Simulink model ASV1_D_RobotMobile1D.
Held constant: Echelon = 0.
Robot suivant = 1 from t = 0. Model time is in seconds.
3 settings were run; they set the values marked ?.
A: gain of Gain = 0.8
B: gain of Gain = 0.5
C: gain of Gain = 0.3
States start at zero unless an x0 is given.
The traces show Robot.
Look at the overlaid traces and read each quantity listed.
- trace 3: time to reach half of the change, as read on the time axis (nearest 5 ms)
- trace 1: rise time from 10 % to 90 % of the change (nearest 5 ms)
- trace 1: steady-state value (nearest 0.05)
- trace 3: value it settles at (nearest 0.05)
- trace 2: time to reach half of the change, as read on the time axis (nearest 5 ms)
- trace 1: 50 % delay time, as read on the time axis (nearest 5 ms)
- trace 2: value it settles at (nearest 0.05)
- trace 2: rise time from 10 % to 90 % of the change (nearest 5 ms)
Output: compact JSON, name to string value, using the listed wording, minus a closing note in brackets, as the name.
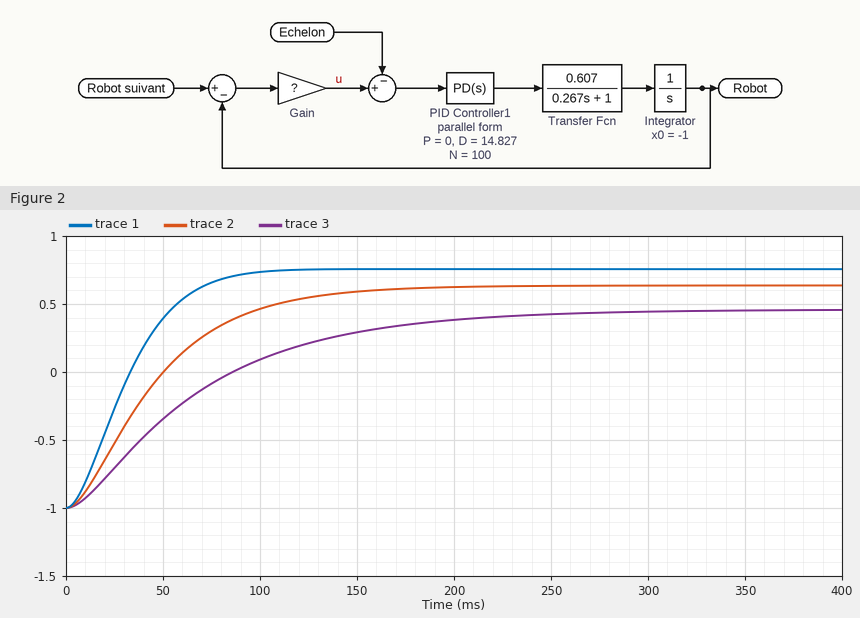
{"trace 3: time to reach half of the change, as read on the time axis": "55 ms", "trace 1: rise time from 10 % to 90 % of the change": "55 ms", "trace 1: steady-state value": "0.75", "trace 3: value it settles at": "0.45", "trace 2: time to reach half of the change, as read on the time axis": "40 ms", "trace 1: 50 % delay time, as read on the time axis": "30 ms", "trace 2: value it settles at": "0.65", "trace 2: rise time from 10 % to 90 % of the change": "90 ms"}
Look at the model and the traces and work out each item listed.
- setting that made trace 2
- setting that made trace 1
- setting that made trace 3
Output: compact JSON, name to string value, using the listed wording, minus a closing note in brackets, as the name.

{"setting that made trace 2": "B", "setting that made trace 1": "A", "setting that made trace 3": "C"}
